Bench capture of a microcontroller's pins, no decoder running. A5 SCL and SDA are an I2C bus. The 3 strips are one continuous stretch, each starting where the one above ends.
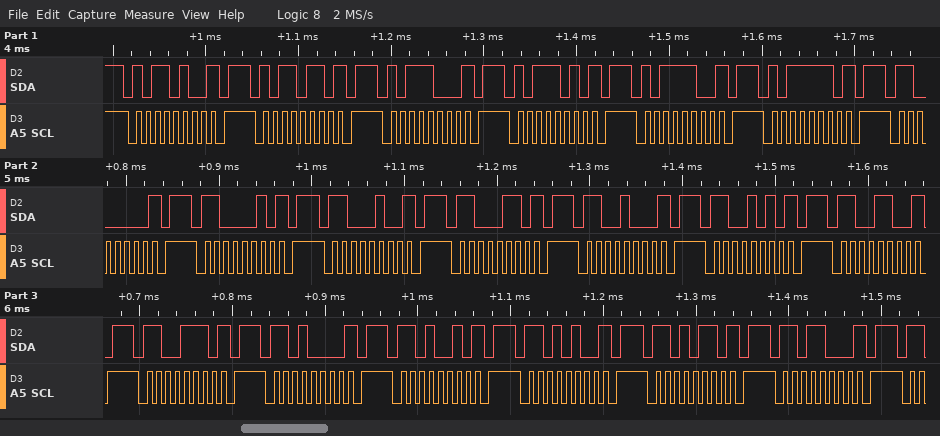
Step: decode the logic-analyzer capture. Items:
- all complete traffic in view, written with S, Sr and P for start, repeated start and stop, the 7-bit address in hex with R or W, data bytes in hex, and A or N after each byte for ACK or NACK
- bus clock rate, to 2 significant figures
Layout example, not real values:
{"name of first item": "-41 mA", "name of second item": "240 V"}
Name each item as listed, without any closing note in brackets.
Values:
{"all complete traffic in view, written with S, Sr and P for start, repeated start and stop, the 7-bit address in hex with R or W, data bytes in hex, and A or N after each byte for ACK or NACK": "S 5AW N P S 5BW N P S 5CW N P S 5DW N P S 5EW N P S 5FW N P S 60W N P S 61W N P S 62W N P S 63W N P S 64W N P S 65W N P S 66W N P S 67W N P S 68W N P S 69W N P S 6AW N P S 6BW N P S 6CW N P", "bus clock rate, to 2 significant figures": "100 kHz"}
